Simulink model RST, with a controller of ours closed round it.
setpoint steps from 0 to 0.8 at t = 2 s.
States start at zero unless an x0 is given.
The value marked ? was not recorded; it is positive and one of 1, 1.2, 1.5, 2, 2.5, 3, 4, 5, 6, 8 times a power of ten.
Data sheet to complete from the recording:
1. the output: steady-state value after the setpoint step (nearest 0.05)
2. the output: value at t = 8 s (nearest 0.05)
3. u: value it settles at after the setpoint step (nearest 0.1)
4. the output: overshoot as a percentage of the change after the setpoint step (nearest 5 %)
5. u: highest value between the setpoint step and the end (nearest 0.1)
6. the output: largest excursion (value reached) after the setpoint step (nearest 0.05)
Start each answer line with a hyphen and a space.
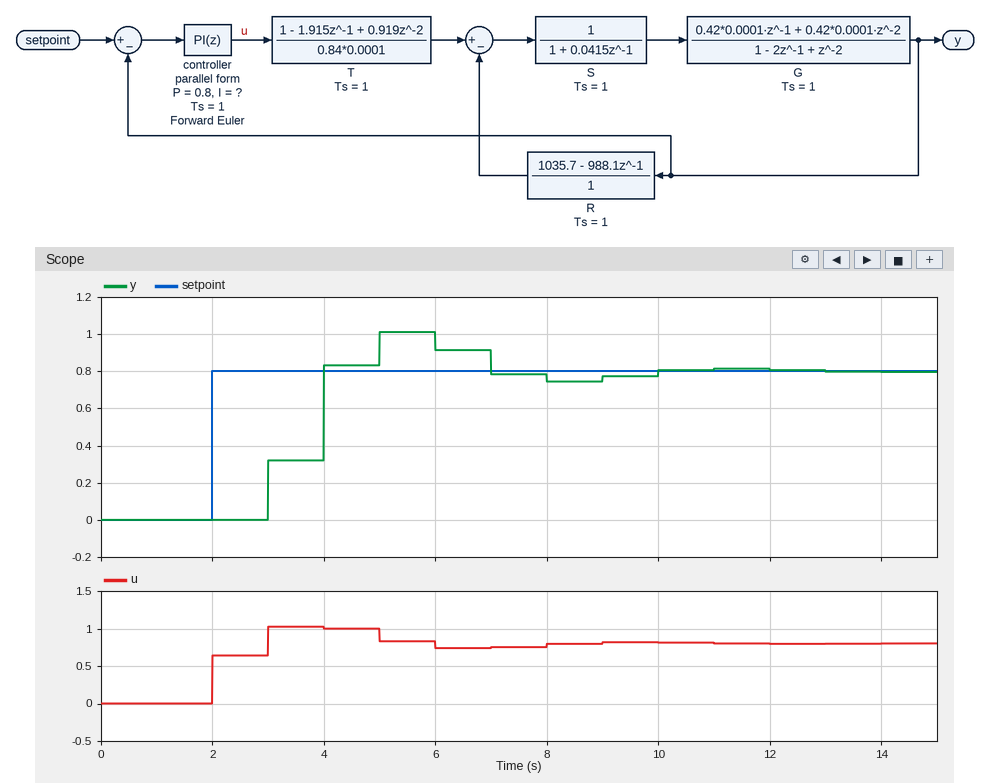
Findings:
- 0.80
- 0.75
- 0.8
- 25 %
- 1.0
- 1.00
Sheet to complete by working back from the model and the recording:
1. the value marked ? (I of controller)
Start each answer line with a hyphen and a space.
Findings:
- 0.8
